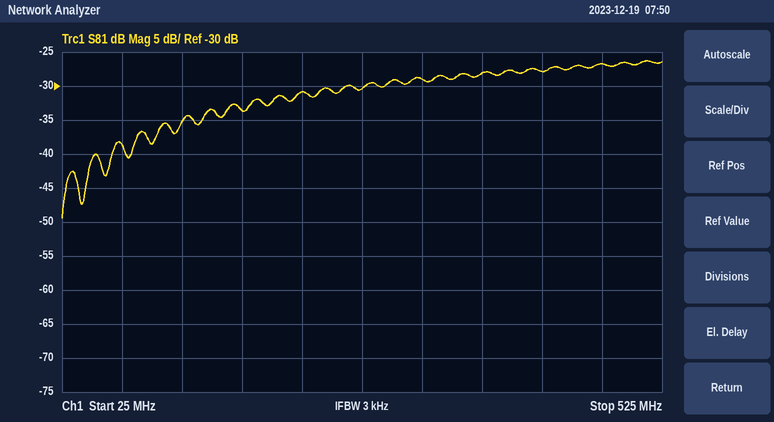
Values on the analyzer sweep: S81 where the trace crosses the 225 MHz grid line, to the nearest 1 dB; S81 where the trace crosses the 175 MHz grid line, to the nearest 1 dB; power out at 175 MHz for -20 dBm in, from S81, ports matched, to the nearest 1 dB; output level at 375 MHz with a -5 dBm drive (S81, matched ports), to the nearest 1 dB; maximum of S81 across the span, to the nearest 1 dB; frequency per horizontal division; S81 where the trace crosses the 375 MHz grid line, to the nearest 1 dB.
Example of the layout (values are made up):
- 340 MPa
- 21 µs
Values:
- -31 dB
- -34 dB
- -54 dBm
- -33 dBm
- -26 dB
- 50 MHz
- -28 dB
